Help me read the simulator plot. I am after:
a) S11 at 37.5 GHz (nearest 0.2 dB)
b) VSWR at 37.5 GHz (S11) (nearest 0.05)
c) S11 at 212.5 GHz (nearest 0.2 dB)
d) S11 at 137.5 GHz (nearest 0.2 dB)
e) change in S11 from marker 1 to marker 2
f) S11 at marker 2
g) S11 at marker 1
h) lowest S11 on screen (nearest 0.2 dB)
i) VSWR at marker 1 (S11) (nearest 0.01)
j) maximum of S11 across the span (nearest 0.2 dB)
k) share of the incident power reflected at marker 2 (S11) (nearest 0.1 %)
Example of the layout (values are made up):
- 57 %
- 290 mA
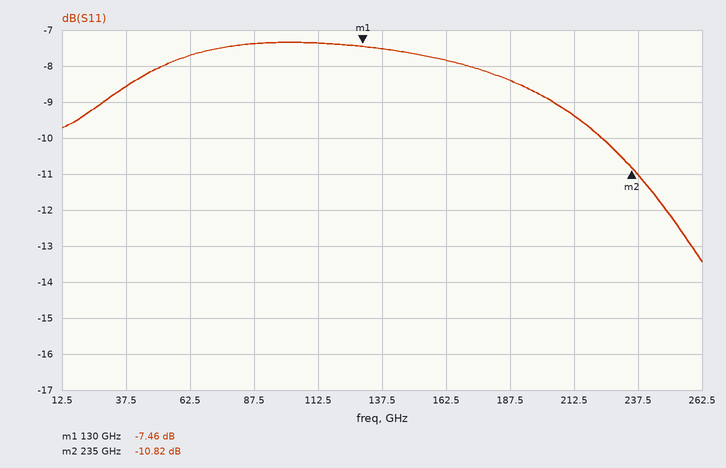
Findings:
- -8.6 dB
- 2.20
- -9.4 dB
- -7.6 dB
- -3.36 dB
- -10.82 dB
- -7.46 dB
- -13.4 dB
- 2.47
- -7.4 dB
- 8.3 %
